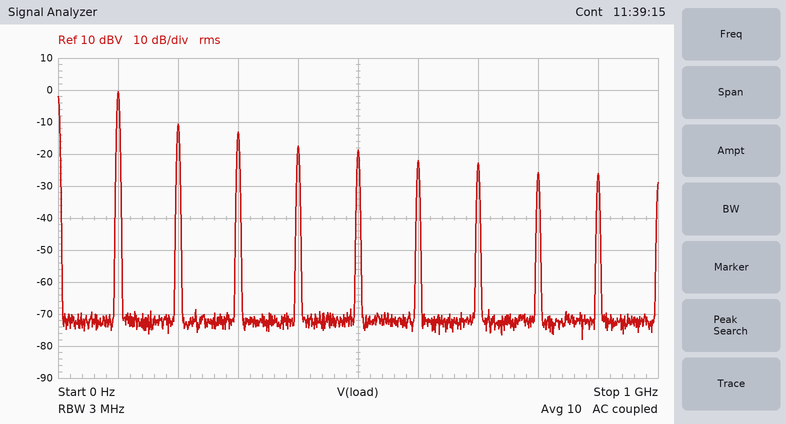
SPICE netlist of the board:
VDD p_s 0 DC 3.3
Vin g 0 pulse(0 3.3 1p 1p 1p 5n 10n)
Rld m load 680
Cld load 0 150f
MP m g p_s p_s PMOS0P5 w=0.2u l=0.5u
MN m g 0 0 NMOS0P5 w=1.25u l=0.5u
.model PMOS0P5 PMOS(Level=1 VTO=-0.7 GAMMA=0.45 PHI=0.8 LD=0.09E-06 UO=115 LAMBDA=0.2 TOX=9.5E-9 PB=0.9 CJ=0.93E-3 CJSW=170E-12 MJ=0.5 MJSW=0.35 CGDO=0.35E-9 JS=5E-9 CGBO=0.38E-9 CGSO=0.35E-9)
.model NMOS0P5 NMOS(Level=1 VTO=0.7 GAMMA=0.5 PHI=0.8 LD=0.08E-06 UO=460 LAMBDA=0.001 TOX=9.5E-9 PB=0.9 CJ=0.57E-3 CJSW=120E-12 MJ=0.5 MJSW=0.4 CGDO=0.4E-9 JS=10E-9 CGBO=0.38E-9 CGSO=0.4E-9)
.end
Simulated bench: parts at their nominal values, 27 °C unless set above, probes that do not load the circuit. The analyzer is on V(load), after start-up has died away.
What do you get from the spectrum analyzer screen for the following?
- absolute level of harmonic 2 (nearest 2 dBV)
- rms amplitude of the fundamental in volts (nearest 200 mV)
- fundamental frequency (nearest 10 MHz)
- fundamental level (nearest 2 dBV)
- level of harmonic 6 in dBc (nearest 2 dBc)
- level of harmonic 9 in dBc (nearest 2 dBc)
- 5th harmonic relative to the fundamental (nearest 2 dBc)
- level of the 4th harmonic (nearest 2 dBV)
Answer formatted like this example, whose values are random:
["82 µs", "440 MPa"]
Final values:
["-10 dBV", "1.0 V", "100 MHz", "0 dBV", "-22 dBc", "-26 dBc", "-18 dBc", "-18 dBV"]
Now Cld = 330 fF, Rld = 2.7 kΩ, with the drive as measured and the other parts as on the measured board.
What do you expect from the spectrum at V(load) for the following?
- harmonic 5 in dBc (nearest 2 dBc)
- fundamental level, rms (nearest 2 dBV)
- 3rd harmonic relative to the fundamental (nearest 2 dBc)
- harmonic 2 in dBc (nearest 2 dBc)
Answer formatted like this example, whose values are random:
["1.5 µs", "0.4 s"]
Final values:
["-24 dBc", "-6 dBV", "-16 dBc", "-14 dBc"]
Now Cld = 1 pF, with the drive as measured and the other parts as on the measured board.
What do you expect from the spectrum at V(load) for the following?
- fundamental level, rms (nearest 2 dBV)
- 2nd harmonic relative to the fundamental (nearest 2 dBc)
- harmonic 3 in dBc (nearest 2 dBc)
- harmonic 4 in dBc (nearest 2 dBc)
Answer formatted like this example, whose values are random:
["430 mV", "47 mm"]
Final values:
["-14 dBV", "-14 dBc", "-16 dBc", "-26 dBc"]
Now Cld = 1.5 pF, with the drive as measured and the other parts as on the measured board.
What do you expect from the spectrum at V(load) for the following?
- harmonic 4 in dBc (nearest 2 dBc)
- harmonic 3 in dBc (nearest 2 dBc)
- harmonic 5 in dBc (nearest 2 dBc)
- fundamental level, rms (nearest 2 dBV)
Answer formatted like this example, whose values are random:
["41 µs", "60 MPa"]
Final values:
["-28 dBc", "-18 dBc", "-26 dBc", "-18 dBV"]
